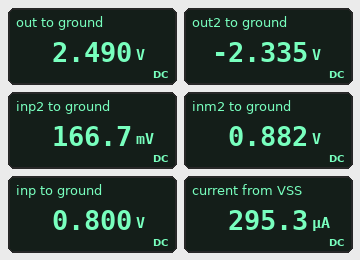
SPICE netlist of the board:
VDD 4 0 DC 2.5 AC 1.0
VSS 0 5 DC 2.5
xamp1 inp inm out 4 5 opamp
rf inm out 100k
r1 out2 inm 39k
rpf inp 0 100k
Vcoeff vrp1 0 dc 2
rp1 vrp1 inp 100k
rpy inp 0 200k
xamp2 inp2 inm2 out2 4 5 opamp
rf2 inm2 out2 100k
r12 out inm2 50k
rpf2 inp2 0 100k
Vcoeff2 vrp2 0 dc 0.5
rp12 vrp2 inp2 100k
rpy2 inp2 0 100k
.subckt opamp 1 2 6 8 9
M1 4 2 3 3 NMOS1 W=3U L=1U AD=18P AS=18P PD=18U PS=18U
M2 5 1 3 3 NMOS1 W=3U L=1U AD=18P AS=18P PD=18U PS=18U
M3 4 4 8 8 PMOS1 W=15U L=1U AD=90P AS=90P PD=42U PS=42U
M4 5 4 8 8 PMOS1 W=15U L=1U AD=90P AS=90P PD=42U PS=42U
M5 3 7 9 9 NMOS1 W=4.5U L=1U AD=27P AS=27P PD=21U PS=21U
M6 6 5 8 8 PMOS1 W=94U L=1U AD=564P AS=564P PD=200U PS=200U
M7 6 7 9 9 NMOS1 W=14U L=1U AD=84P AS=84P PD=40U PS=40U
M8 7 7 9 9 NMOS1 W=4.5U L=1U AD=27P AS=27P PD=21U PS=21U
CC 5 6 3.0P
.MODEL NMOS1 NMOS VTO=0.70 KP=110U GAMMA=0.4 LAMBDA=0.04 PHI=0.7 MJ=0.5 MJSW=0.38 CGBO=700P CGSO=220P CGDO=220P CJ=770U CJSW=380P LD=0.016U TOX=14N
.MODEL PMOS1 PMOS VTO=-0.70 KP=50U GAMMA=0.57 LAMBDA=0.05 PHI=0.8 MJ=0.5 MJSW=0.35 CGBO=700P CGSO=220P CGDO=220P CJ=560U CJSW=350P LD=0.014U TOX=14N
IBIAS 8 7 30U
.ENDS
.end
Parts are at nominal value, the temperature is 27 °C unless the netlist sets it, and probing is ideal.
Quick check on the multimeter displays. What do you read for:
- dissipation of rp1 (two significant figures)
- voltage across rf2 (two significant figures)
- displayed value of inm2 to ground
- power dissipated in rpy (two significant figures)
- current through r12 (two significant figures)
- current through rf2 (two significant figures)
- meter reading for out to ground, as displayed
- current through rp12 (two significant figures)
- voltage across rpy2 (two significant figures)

14 µW
3.2 V
0.882 V
3.2 µW
32 µA
32 µA
2.490 V
3.3 µA
170 mV
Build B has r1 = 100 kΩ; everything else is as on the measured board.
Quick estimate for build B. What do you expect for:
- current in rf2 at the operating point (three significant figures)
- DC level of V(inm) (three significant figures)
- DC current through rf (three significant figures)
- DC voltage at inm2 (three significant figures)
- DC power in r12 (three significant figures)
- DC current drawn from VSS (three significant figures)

32.4 µA
59.2 mV
24.3 µA
869 mV
52.4 µW
286 µA
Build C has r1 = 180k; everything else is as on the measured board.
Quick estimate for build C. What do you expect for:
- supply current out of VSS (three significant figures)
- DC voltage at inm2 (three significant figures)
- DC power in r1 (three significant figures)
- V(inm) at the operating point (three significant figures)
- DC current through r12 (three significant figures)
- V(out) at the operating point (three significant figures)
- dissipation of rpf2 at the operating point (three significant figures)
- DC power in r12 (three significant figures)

280 µA
859 mV
54.5 µW
743 mV
32.5 µA
2.48 V
278 nW
52.7 µW
